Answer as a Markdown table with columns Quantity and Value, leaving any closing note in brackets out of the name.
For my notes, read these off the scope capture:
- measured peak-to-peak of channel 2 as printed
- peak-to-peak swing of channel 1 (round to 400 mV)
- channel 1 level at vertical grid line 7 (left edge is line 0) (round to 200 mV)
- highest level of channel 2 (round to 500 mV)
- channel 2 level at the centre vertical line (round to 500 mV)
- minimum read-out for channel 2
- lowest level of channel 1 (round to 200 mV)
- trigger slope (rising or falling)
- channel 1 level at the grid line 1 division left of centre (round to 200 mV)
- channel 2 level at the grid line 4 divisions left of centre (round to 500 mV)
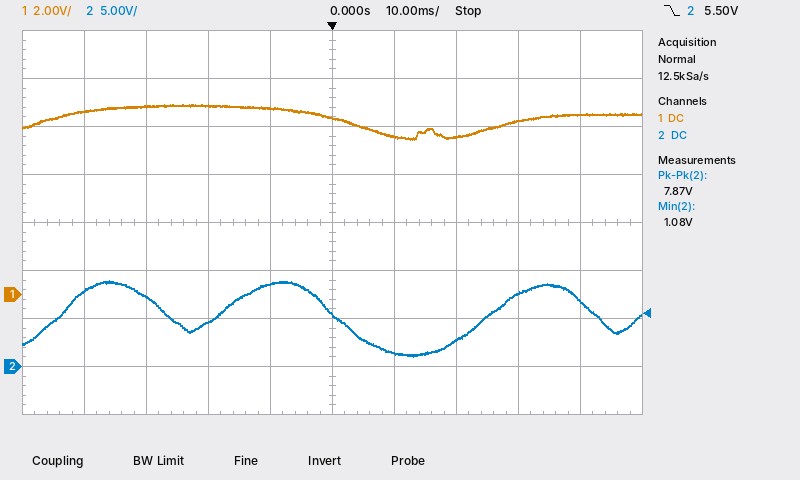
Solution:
| Quantity | Value |
|---|---|
| measured peak-to-peak of channel 2 as printed | 7.87 V |
| peak-to-peak swing of channel 1 | 1.6 V |
| channel 1 level at vertical grid line 7 (left edge is line 0) | 6.6 V |
| highest level of channel 2 | 9.0 V |
| channel 2 level at the centre vertical line | 5.5 V |
| minimum read-out for channel 2 | 1.08 V |
| lowest level of channel 1 | 6.4 V |
| trigger slope | falling |
| channel 1 level at the grid line 1 division left of centre | 7.8 V |
| channel 2 level at the grid line 4 divisions left of centre | 8.0 V |
